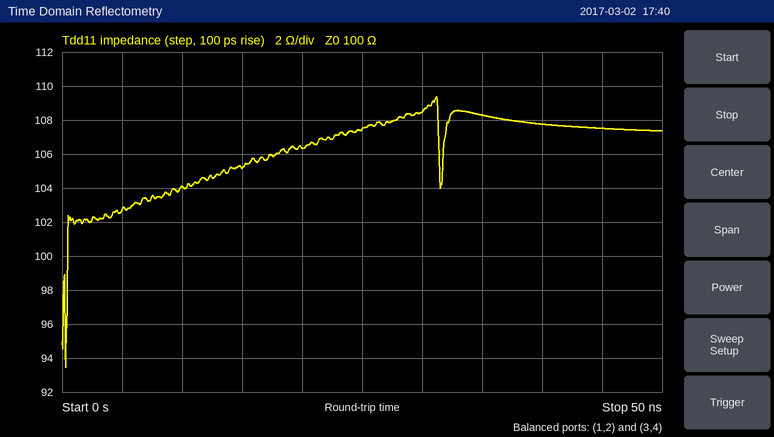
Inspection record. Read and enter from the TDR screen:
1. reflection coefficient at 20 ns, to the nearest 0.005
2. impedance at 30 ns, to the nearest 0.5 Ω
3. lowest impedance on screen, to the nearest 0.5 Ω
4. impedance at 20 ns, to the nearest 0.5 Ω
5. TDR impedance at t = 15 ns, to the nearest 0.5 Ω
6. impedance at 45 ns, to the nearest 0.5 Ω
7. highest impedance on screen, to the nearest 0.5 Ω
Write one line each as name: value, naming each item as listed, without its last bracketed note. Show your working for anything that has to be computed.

reflection coefficient at 20 ns, to the nearest 0.005: (106.5 − 100)/(106.5 + 100) ≈ +0.0315, so +0.030 to the nearest 0.005
impedance at 30 ns, to the nearest 0.5 Ω: 108.5 Ω
lowest impedance on screen, to the nearest 0.5 Ω: 93.5 Ω
impedance at 20 ns, to the nearest 0.5 Ω: 106.5 Ω
TDR impedance at t = 15 ns, to the nearest 0.5 Ω: 105.0 Ω
impedance at 45 ns, to the nearest 0.5 Ω: 107.5 Ω
highest impedance on screen, to the nearest 0.5 Ω: 109.5 Ω
